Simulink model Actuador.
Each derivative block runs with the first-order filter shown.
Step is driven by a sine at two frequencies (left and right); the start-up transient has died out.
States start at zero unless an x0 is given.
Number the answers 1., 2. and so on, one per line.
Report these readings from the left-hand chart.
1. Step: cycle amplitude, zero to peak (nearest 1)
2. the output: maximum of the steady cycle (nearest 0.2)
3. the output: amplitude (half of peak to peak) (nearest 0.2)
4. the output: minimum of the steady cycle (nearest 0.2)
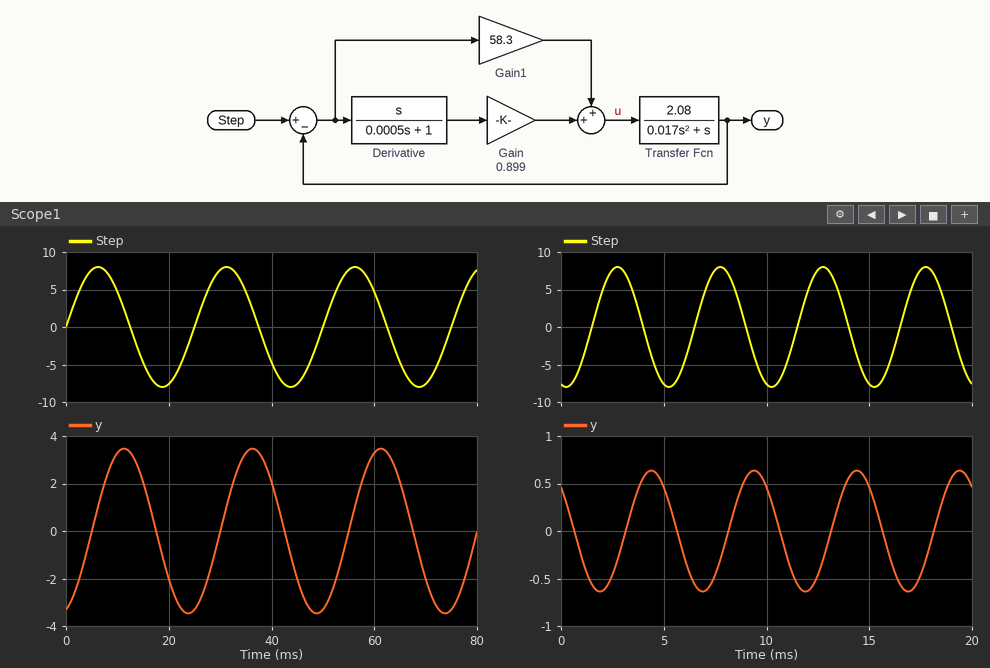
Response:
1. 8
2. 3.4
3. 3.4
4. -3.4
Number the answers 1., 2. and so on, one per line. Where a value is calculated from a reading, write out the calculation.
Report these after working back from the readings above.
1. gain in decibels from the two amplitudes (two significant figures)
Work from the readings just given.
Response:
1. 20 log10(3.4 / 8) = -7.4 dB
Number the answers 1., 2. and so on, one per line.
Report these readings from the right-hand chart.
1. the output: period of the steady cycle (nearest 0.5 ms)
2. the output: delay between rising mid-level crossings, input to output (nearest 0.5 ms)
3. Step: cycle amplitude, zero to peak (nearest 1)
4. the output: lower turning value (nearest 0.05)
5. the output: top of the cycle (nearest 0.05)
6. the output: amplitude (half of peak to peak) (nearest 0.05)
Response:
1. 5.0 ms
2. 1.5 ms
3. 8
4. -0.65
5. 0.65
6. 0.65
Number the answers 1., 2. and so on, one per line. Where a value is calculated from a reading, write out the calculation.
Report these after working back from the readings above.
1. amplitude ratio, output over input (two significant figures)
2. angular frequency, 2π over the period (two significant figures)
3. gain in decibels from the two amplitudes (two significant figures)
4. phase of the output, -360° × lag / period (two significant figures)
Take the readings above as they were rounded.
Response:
1. 0.65 / 8 = 0.081
2. 2π / 5 = 1.3 rad/ms
3. 20 log10(0.65 / 8) = -22 dB
4. -360 × 1.5 / 5 = -110°
